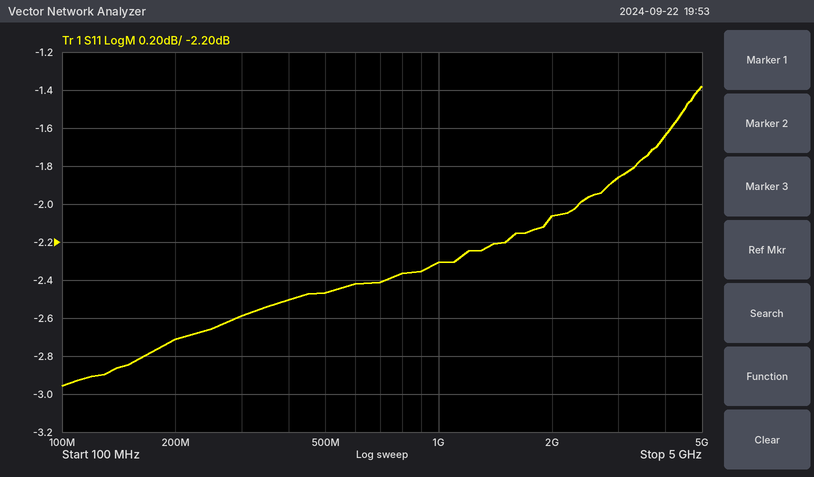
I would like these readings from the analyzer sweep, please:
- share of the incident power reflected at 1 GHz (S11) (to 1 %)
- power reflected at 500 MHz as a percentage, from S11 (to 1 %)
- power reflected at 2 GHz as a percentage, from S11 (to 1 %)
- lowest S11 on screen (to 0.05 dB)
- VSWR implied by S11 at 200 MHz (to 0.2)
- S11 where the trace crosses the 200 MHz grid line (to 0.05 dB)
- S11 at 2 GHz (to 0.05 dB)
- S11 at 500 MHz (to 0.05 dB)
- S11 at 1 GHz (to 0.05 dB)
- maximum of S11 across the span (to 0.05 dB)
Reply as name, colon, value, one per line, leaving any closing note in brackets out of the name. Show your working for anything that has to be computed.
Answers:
share of the incident power reflected at 1 GHz (S11): 10^(-2.3/10) ≈ 59 %
power reflected at 500 MHz as a percentage, from S11: 10^(-2.45/10) ≈ 57 %
power reflected at 2 GHz as a percentage, from S11: 10^(-2.05/10) ≈ 62 %
lowest S11 on screen: -2.95 dB
VSWR implied by S11 at 200 MHz: |Γ| = 10^(-2.7/20) = 0.7328; VSWR = (1 + 0.7328)/(1 − 0.7328) ≈ 6.49, so 6.4 to the nearest 0.2
S11 where the trace crosses the 200 MHz grid line: -2.70 dB
S11 at 2 GHz: -2.05 dB
S11 at 500 MHz: -2.45 dB
S11 at 1 GHz: -2.30 dB
maximum of S11 across the span: -1.40 dB
